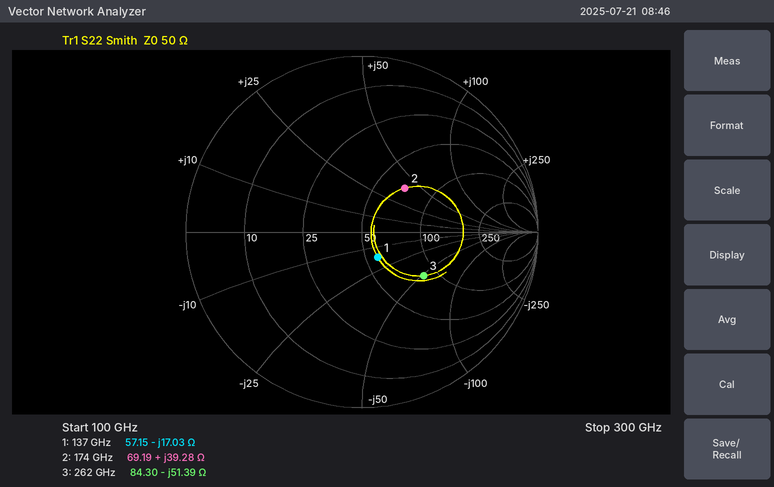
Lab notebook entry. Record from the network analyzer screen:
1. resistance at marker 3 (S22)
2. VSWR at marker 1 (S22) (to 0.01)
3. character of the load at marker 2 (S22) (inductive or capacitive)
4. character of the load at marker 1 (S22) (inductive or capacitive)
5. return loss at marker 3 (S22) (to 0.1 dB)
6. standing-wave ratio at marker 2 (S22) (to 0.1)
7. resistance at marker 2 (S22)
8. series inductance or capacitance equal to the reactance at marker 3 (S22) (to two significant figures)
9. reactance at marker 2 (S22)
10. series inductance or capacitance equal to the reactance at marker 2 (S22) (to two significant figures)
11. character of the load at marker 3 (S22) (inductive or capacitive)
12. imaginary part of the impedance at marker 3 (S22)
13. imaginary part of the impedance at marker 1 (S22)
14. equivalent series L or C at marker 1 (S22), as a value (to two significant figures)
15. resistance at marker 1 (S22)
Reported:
84.30 Ω
1.41
inductive
capacitive
7.3 dB
2.1
69.19 Ω
12 fF
+39.28 Ω
36 pH
capacitive
-51.39 Ω
-17.03 Ω
68 fF
57.15 Ω
